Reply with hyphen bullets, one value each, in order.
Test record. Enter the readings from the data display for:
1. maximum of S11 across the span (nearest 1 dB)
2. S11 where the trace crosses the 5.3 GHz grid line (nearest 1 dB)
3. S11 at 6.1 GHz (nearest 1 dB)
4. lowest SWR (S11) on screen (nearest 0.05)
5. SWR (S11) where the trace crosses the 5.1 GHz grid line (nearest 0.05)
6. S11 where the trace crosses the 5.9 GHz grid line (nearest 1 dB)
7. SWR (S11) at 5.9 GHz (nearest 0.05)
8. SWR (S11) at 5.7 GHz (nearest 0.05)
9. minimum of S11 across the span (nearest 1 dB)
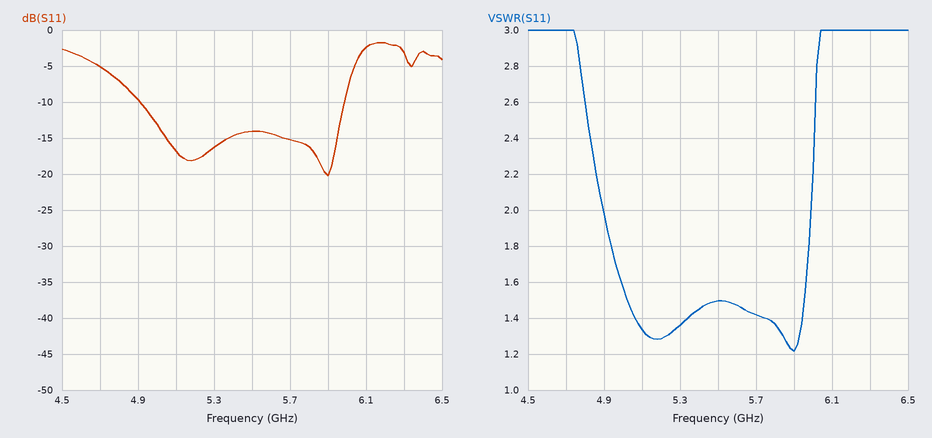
- -2 dB
- -16 dB
- -2 dB
- 1.20
- 1.35
- -20 dB
- 1.20
- 1.40
- -20 dB
